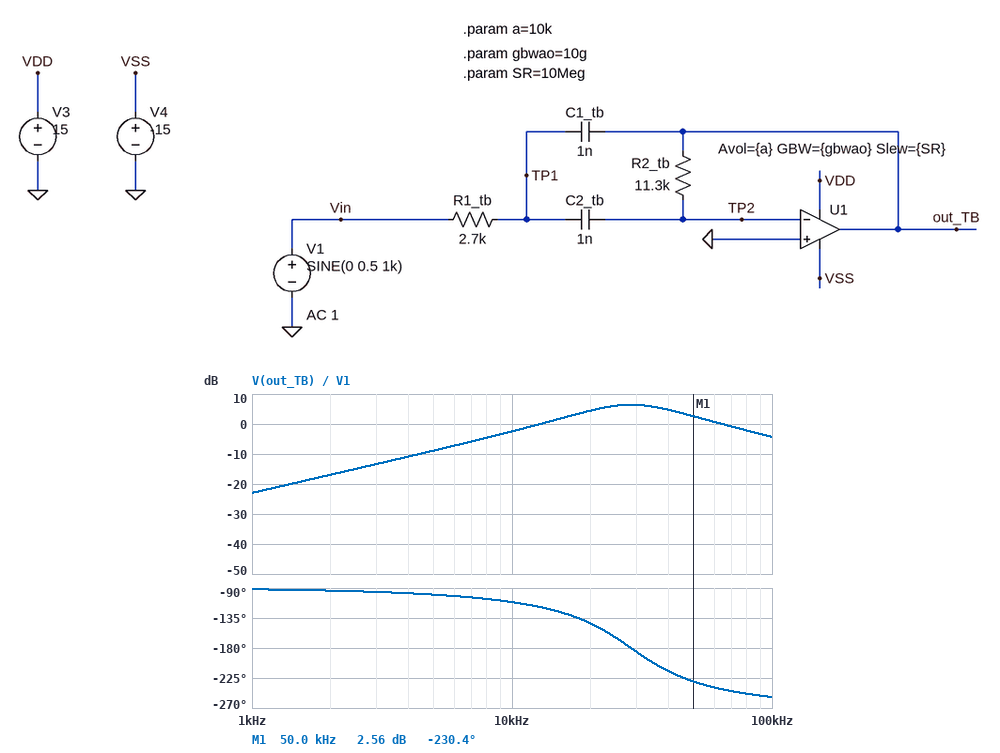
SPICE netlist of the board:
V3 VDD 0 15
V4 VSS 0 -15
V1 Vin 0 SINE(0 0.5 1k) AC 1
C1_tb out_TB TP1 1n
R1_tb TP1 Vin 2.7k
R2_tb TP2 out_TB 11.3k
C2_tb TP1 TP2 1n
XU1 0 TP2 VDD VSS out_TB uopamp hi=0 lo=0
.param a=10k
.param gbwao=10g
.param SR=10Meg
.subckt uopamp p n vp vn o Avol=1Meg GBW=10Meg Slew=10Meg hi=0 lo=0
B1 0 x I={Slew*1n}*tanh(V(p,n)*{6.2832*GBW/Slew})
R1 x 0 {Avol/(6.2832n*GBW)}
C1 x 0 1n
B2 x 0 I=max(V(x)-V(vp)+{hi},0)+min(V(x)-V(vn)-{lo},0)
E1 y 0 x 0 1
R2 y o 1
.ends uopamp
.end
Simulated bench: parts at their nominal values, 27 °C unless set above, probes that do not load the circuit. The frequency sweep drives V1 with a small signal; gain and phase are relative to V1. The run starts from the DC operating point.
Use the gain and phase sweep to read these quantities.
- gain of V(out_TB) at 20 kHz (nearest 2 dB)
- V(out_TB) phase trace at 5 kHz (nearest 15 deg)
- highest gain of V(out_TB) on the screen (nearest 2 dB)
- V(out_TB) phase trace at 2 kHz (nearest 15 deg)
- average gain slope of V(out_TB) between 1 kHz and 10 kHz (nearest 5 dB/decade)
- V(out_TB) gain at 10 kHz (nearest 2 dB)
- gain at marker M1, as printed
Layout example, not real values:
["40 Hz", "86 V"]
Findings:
["4 dB", "-105 deg", "6 dB", "-90 deg", "20 dB/decade", "-2 dB", "2.56 dB"]
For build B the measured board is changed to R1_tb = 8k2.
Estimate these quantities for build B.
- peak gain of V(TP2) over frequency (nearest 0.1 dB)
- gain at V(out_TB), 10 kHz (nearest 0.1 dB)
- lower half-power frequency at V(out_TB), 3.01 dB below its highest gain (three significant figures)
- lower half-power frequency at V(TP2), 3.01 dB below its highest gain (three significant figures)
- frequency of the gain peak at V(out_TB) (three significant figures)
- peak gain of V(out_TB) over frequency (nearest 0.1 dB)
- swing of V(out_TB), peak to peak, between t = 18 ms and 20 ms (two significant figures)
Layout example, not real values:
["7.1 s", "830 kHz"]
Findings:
["-54.3 dB", "-4.6 dB", "7.63 kHz", "20.5 kHz", "16.5 kHz", "-3.2 dB", "71 mV"]
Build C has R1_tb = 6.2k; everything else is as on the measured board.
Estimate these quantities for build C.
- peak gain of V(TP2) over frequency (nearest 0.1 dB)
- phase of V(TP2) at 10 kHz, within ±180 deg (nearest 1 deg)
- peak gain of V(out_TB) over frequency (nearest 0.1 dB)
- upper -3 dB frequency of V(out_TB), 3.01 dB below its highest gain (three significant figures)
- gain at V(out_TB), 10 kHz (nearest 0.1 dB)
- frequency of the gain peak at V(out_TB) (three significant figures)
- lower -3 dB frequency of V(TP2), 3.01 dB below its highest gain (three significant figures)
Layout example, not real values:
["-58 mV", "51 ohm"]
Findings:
["-51.8 dB", "133 deg", "-0.8 dB", "37.7 kHz", "-3.5 dB", "19.0 kHz", "19.9 kHz"]
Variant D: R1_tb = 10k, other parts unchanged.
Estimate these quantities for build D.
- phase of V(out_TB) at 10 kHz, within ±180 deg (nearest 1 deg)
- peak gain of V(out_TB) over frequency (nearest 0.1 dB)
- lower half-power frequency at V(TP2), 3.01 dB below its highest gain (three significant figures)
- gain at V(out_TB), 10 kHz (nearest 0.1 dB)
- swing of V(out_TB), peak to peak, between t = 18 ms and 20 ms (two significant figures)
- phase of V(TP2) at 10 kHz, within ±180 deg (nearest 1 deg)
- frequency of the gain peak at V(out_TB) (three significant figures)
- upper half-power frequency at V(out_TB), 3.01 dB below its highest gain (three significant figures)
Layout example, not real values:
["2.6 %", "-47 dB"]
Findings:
["-156 deg", "-5.0 dB", "21.2 kHz", "-5.7 dB", "71 mV", "114 deg", "15.0 kHz", "34.6 kHz"]
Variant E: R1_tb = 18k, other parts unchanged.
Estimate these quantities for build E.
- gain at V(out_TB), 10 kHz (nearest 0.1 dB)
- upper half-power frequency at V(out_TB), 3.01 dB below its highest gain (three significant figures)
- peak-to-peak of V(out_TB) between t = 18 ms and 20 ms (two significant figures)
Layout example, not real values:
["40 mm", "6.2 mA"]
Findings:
["-10.1 dB", "32.0 kHz", "70 mV"]
